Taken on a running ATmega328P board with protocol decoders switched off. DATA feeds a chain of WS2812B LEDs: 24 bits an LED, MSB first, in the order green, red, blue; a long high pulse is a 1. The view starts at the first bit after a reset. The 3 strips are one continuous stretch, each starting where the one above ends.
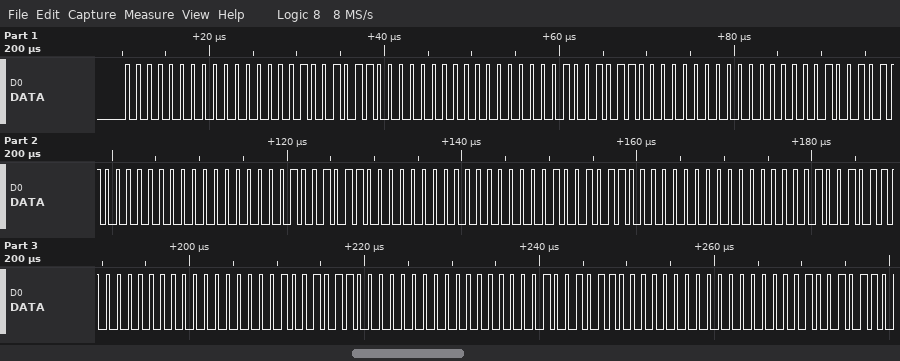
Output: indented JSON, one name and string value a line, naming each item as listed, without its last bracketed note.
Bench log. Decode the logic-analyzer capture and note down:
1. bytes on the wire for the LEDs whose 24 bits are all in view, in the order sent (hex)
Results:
{
  "bytes on the wire for the LEDs whose 24 bits are all in view, in the order sent": "00 00 96 00 00 96 00 00 96 00 00 96 00 00 96 00 00 96 00 00 96 00 00 96 00 00 96"
}
